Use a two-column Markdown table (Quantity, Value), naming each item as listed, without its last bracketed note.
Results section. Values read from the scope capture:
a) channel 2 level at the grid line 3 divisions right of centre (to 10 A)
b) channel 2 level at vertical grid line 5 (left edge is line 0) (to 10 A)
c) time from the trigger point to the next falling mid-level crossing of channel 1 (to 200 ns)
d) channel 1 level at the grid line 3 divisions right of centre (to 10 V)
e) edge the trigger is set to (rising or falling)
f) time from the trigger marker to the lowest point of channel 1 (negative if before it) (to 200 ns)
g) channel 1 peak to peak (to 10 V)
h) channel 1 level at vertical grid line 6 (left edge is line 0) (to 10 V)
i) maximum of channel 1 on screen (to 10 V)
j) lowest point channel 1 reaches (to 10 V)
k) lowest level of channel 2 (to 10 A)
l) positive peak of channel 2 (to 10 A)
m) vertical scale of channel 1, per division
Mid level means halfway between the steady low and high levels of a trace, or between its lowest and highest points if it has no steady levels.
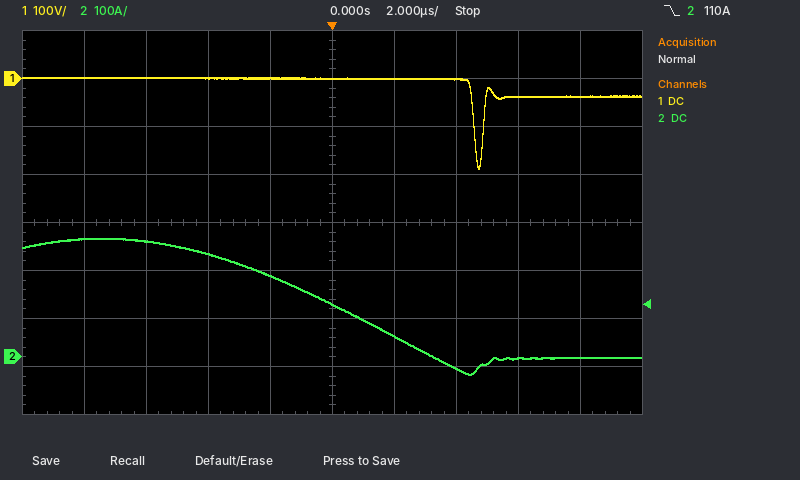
| Quantity | Value |
|---|---|
| channel 2 level at the grid line 3 divisions right of centre | 0 A |
| channel 2 level at vertical grid line 5 (left edge is line 0) | 110 A |
| time from the trigger point to the next falling mid-level crossing of channel 1 | 4.6 µs |
| channel 1 level at the grid line 3 divisions right of centre | -40 V |
| edge the trigger is set to | falling |
| time from the trigger marker to the lowest point of channel 1 (negative if before it) | +4.8 µs |
| channel 1 peak to peak | 190 V |
| channel 1 level at vertical grid line 6 (left edge is line 0) | 0 V |
| maximum of channel 1 on screen | 0 V |
| lowest point channel 1 reaches | -190 V |
| lowest level of channel 2 | -40 A |
| positive peak of channel 2 | 250 A |
| vertical scale of channel 1, per division | 100 V |
